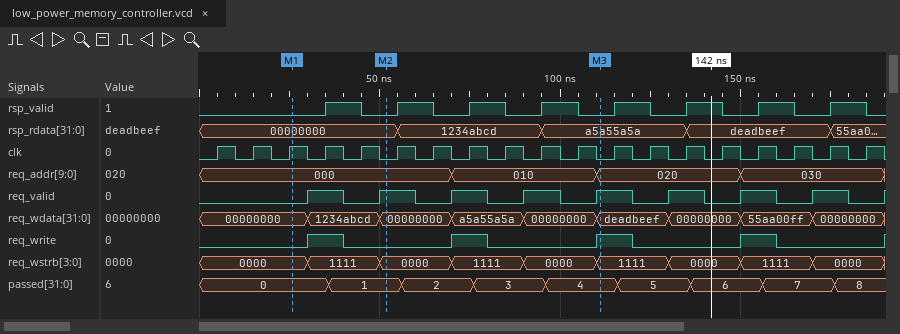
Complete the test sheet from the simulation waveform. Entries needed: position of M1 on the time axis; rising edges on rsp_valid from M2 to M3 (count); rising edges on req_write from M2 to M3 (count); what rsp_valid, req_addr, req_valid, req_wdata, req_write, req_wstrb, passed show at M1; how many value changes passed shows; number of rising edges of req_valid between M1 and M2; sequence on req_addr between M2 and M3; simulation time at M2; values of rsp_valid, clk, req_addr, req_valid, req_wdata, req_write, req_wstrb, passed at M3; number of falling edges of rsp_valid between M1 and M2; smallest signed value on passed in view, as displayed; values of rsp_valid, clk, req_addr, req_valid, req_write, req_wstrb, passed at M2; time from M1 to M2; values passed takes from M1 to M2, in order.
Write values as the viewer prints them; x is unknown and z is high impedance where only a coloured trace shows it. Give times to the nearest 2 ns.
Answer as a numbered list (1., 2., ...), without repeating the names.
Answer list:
1. 26 ns
2. 3
3. 2
4. rsp_valid=0, req_addr=000, req_valid=0, req_wdata=00000000, req_write=0, req_wstrb=0000, passed=0
5. 8
6. 2
7. 000, 010, 020
8. 52 ns
9. rsp_valid=0, clk=0, req_addr=020, req_valid=1, req_wdata=deadbeef, req_write=1, req_wstrb=1111, passed=4
10. 1
11. 0
12. rsp_valid=0, clk=0, req_addr=000, req_valid=1, req_write=0, req_wstrb=0000, passed=1
13. 26 ns
14. 0, 1
